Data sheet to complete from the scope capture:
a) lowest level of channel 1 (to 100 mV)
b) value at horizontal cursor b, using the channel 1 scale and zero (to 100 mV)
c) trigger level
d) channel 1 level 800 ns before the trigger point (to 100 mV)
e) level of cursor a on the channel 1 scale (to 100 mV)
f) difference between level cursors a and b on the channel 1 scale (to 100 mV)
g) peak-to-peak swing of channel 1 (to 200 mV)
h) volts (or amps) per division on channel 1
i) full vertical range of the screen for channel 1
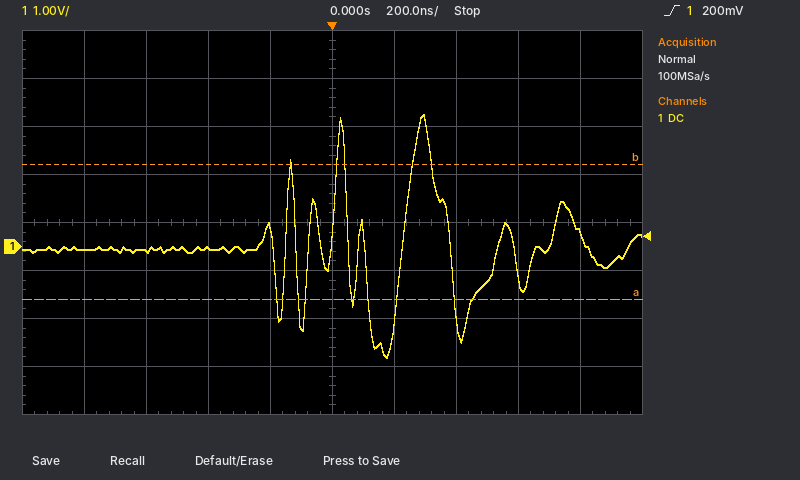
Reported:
-2.3 V
1.7 V
200 mV
-100 mV
-1.1 V
2.8 V
5.0 V
1 V
8 V
